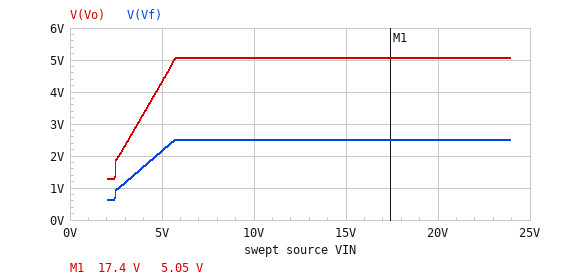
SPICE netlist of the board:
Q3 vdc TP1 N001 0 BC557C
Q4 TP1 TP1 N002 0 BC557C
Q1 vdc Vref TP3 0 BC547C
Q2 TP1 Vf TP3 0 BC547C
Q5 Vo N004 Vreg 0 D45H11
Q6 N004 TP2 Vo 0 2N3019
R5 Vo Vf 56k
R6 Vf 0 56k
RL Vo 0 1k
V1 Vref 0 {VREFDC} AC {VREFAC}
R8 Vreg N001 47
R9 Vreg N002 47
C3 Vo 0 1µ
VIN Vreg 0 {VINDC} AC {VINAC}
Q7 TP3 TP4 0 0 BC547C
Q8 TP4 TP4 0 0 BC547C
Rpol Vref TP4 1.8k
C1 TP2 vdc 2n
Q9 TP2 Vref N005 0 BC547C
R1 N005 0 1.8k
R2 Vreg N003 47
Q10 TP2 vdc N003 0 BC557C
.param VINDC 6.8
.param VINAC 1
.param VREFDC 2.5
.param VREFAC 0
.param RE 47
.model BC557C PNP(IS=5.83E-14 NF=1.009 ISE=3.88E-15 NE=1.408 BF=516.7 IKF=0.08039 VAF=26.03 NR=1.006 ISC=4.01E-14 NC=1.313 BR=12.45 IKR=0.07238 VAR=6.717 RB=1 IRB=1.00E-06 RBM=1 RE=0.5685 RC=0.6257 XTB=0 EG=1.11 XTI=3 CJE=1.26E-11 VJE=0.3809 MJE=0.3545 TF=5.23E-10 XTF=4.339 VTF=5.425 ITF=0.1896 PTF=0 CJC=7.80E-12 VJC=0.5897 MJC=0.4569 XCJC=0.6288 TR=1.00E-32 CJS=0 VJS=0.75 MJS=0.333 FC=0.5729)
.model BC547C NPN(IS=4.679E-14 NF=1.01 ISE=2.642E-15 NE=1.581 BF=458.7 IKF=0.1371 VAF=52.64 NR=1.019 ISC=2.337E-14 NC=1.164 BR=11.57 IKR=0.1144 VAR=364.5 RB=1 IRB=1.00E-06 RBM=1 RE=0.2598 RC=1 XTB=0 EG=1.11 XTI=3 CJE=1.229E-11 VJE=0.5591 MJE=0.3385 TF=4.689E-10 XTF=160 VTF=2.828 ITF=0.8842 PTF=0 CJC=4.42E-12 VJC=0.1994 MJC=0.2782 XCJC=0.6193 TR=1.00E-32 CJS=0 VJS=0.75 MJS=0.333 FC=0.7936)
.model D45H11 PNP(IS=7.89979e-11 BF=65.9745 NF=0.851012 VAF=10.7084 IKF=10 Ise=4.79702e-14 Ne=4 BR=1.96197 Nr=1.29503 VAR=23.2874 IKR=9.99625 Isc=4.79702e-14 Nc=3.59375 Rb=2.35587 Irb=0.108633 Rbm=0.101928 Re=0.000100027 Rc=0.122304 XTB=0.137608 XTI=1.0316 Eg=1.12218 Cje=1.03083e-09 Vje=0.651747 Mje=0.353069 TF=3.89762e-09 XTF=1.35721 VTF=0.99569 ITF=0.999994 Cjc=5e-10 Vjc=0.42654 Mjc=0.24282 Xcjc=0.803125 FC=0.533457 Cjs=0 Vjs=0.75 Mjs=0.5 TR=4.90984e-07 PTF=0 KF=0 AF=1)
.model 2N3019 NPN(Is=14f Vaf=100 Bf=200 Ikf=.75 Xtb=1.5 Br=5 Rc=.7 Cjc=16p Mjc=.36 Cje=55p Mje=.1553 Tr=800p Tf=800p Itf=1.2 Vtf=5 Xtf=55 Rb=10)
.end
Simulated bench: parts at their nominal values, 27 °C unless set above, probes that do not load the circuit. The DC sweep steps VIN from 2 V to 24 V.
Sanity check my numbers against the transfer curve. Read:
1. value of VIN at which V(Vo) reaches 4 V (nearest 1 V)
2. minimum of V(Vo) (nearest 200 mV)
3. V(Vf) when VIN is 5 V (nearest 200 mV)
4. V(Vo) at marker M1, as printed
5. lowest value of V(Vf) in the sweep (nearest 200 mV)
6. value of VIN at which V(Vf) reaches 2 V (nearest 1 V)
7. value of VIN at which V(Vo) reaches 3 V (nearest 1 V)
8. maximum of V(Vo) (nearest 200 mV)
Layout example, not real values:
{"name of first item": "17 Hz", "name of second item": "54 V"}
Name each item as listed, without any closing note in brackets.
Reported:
{"value of VIN at which V(Vo) reaches 4 V": "5 V", "minimum of V(Vo)": "1.2 V", "V(Vf) when VIN is 5 V": "2.2 V", "V(Vo) at marker M1, as printed": "5.05 V", "lowest value of V(Vf) in the sweep": "600 mV", "value of VIN at which V(Vf) reaches 2 V": "5 V", "value of VIN at which V(Vo) reaches 3 V": "4 V", "maximum of V(Vo)": "5.0 V"}
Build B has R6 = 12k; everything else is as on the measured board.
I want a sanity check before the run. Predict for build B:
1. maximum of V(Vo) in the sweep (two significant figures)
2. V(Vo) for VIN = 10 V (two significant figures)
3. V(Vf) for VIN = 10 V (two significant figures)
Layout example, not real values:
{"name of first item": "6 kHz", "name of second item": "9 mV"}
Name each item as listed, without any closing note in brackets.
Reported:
{"maximum of V(Vo) in the sweep": "14 V", "V(Vo) for VIN = 10 V": "9.3 V", "V(Vf) for VIN = 10 V": "1.6 V"}
